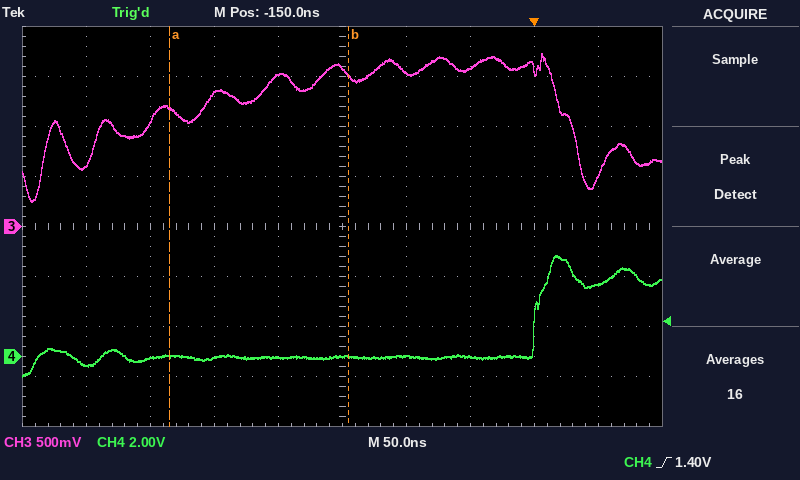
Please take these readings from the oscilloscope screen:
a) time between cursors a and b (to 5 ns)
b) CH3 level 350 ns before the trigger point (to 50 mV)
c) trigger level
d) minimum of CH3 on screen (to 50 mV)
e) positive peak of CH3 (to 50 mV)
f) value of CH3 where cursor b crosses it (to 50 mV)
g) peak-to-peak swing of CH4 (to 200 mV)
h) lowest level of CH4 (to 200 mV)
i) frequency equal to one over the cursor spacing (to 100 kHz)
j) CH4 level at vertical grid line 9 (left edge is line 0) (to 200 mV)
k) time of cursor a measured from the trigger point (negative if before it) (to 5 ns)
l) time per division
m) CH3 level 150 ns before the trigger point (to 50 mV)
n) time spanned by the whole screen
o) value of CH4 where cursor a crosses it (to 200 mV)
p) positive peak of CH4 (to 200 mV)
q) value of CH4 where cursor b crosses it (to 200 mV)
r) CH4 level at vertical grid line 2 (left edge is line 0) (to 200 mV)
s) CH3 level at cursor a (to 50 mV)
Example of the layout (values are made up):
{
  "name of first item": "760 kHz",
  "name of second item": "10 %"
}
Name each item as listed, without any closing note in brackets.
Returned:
{
  "time between cursors a and b": "140 ns",
  "CH3 level 350 ns before the trigger point": "600 mV",
  "trigger level": "1.40 V",
  "minimum of CH3 on screen": "250 mV",
  "positive peak of CH3": "1.75 V",
  "value of CH3 where cursor b crosses it": "1.50 V",
  "peak-to-peak swing of CH4": "4.8 V",
  "lowest level of CH4": "-800 mV",
  "frequency equal to one over the cursor spacing": "7.1 MHz",
  "CH4 level at vertical grid line 9 (left edge is line 0)": "2.8 V",
  "time of cursor a measured from the trigger point (negative if before it)": "-285 ns",
  "time per division": "50 ns",
  "CH3 level 150 ns before the trigger point": "1.60 V",
  "time spanned by the whole screen": "500 ns",
  "value of CH4 where cursor a crosses it": "0.0 V",
  "positive peak of CH4": "4.0 V",
  "value of CH4 where cursor b crosses it": "0.0 V",
  "CH4 level at vertical grid line 2 (left edge is line 0)": "0.0 V",
  "CH3 level at cursor a": "1.20 V"
}
